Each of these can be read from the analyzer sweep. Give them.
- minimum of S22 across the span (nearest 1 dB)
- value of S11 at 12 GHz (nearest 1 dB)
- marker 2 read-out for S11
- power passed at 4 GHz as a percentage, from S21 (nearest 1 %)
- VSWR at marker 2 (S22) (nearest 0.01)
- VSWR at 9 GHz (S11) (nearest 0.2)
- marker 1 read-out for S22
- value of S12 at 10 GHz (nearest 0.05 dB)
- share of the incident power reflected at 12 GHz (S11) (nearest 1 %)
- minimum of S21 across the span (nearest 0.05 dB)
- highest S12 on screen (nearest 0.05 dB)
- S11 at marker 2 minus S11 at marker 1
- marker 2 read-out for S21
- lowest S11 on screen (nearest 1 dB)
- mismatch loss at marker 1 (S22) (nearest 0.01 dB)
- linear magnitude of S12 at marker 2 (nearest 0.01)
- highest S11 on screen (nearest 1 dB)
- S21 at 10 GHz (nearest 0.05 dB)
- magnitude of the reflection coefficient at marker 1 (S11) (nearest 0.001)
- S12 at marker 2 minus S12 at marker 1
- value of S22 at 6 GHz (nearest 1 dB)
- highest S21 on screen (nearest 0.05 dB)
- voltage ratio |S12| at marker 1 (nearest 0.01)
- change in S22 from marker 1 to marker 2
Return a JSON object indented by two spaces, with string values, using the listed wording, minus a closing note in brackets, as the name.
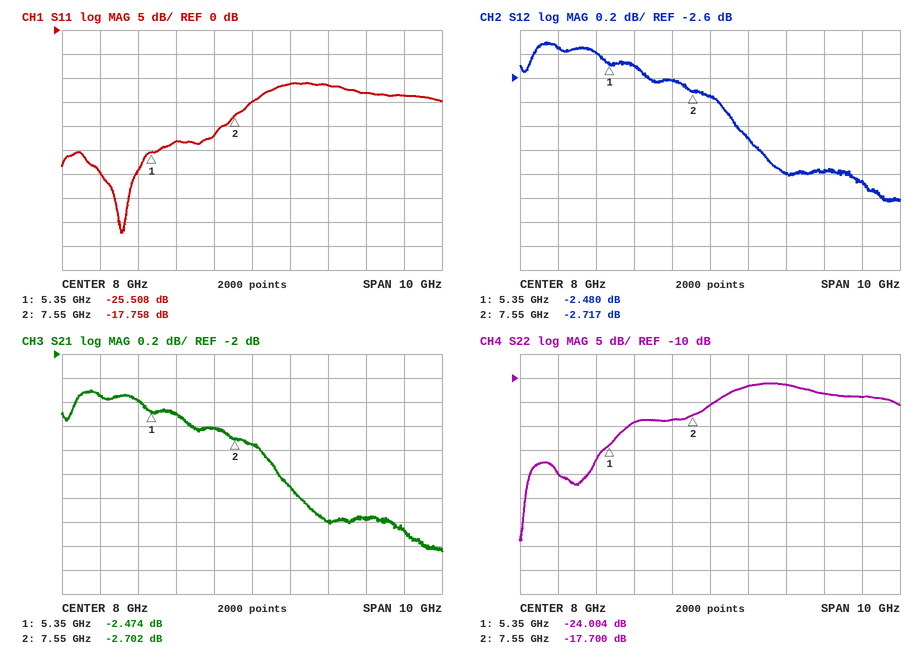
{
  "minimum of S22 across the span": "-44 dB",
  "value of S11 at 12 GHz": "-14 dB",
  "marker 2 read-out for S11": "-17.758 dB",
  "power passed at 4 GHz as a percentage, from S21": "58 %",
  "VSWR at marker 2 (S22)": "1.30",
  "VSWR at 9 GHz (S11)": "1.8",
  "marker 1 read-out for S22": "-24.004 dB",
  "value of S12 at 10 GHz": "-3.40 dB",
  "share of the incident power reflected at 12 GHz (S11)": "4 %",
  "minimum of S21 across the span": "-3.65 dB",
  "highest S12 on screen": "-2.30 dB",
  "S11 at marker 2 minus S11 at marker 1": "7.750 dB",
  "marker 2 read-out for S21": "-2.702 dB",
  "lowest S11 on screen": "-42 dB",
  "mismatch loss at marker 1 (S22)": "0.02 dB",
  "linear magnitude of S12 at marker 2": "0.73",
  "highest S11 on screen": "-11 dB",
  "S21 at 10 GHz": "-3.40 dB",
  "magnitude of the reflection coefficient at marker 1 (S11)": "0.053",
  "S12 at marker 2 minus S12 at marker 1": "-0.237 dB",
  "value of S22 at 6 GHz": "-19 dB",
  "highest S21 on screen": "-2.30 dB",
  "voltage ratio |S12| at marker 1": "0.75",
  "change in S22 from marker 1 to marker 2": "6.304 dB"
}
